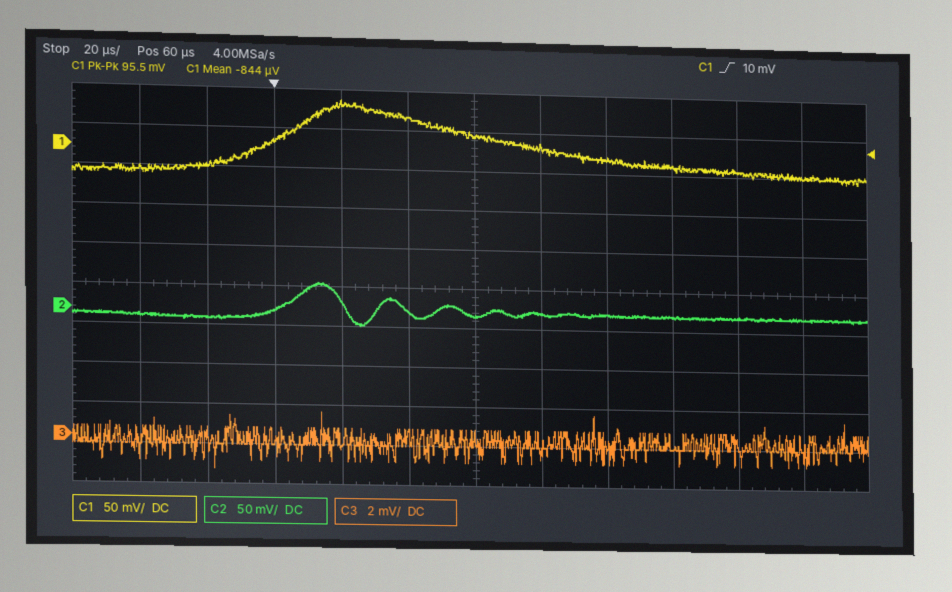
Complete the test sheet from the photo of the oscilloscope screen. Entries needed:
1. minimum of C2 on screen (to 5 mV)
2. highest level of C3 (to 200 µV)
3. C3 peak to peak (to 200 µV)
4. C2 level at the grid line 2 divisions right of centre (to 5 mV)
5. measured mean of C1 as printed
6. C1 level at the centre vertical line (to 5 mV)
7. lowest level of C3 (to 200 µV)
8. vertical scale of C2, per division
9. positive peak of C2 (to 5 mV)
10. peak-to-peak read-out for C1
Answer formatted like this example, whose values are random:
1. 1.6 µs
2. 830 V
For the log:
1. -20 mV
2. 1.2 mV
3. 2.8 mV
4. 0 mV
5. -844 µV
6. 20 mV
7. -1.6 mV
8. 50 mV
9. 35 mV
10. 95.5 mV
